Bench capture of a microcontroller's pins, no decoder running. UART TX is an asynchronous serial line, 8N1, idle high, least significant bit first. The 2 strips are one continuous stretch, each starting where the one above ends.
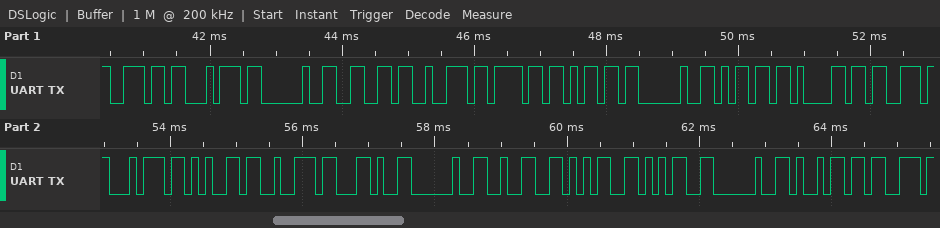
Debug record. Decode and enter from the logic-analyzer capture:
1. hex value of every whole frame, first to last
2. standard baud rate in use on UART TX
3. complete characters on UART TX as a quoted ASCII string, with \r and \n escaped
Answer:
6E 74 20 66 72 6F 6D 20 6D 61 73 74 65 72 2C 20 32 35 35 20 69 73
9600 baud
"nt from master, 255 is"
